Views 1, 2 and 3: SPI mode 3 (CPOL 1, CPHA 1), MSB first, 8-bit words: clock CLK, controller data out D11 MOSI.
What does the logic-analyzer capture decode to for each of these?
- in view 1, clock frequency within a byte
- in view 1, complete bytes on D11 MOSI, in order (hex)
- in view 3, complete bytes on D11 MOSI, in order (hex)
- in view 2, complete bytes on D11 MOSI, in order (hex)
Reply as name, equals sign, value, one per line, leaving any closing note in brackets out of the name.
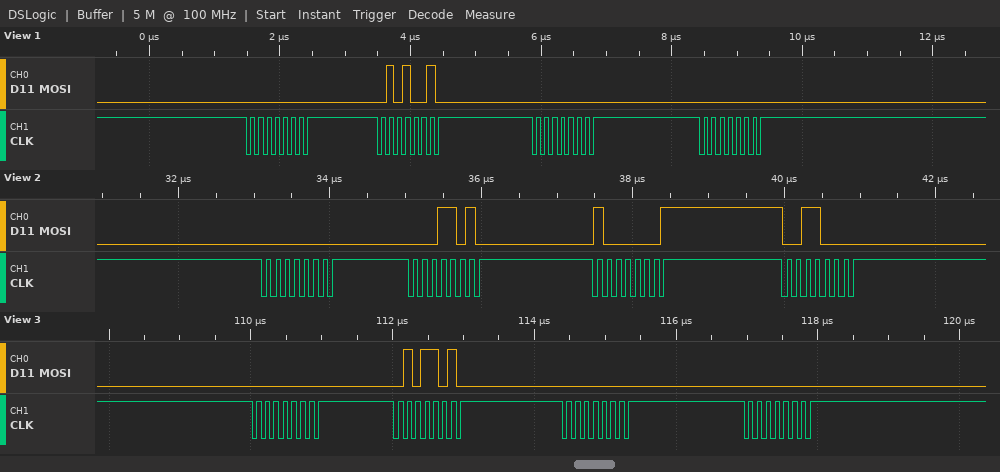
in view 1, clock frequency within a byte = 8 MHz
in view 1, complete bytes on D11 MOSI, in order = 00 52 00 00
in view 3, complete bytes on D11 MOSI, in order = 00 5A 00 00
in view 2, complete bytes on D11 MOSI, in order = 00 1A 81 30
